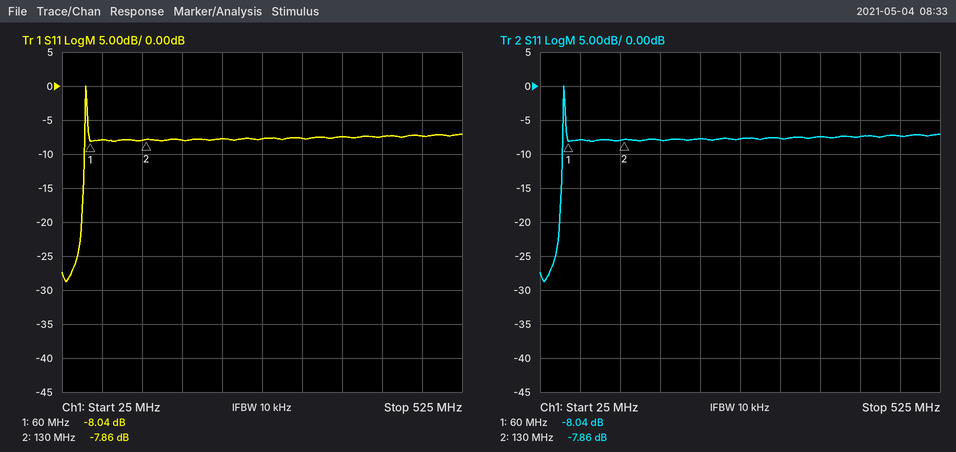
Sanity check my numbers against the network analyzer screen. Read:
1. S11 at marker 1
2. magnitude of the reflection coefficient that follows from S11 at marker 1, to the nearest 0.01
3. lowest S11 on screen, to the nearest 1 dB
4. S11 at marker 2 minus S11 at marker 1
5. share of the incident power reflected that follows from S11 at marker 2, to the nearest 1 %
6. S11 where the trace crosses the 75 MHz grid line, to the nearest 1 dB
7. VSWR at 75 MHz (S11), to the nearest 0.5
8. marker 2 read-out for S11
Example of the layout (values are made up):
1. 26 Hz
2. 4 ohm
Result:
1. -8.04 dB
2. 0.40
3. -29 dB
4. 0.18 dB
5. 16 %
6. -8 dB
7. 2.5
8. -7.86 dB
